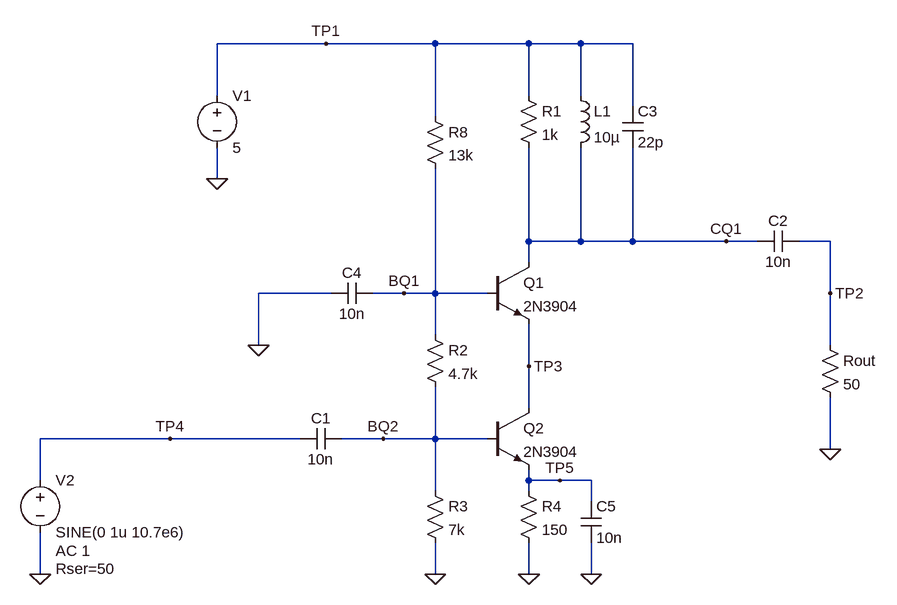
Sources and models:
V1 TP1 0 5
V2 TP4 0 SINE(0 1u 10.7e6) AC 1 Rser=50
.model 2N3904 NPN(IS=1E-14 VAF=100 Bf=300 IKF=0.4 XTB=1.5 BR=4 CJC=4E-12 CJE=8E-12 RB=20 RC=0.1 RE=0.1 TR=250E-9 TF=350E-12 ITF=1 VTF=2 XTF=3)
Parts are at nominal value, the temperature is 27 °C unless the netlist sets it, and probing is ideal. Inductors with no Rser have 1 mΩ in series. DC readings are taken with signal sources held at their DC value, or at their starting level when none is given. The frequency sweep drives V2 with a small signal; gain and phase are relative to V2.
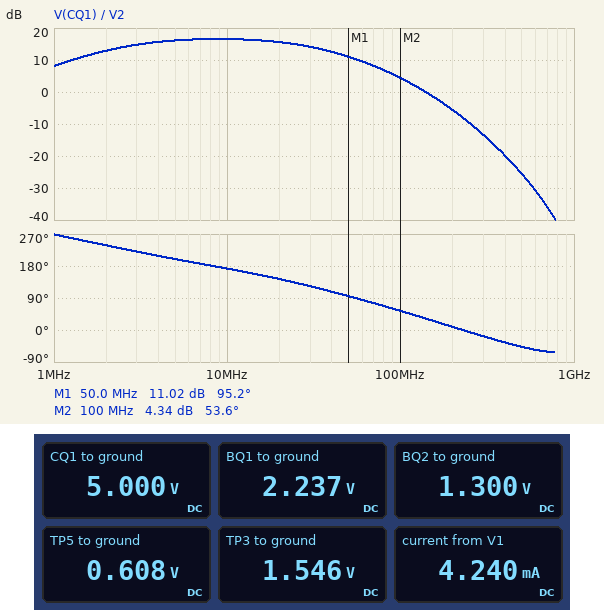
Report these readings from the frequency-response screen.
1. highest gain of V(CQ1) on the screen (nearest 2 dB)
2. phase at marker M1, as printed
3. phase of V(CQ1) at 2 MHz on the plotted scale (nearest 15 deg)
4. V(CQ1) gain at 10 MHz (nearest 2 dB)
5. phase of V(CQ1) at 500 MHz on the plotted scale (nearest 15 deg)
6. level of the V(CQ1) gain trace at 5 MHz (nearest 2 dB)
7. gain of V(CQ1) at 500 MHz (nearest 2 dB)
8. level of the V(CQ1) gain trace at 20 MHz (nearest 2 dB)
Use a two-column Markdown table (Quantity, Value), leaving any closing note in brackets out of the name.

| Quantity | Value |
|---|---|
| highest gain of V(CQ1) on the screen | 16 dB |
| phase at marker M1, as printed | 95.2 deg |
| phase of V(CQ1) at 2 MHz on the plotted scale | 240 deg |
| V(CQ1) gain at 10 MHz | 16 dB |
| phase of V(CQ1) at 500 MHz on the plotted scale | -45 deg |
| level of the V(CQ1) gain trace at 5 MHz | 16 dB |
| gain of V(CQ1) at 500 MHz | -26 dB |
| level of the V(CQ1) gain trace at 20 MHz | 16 dB |
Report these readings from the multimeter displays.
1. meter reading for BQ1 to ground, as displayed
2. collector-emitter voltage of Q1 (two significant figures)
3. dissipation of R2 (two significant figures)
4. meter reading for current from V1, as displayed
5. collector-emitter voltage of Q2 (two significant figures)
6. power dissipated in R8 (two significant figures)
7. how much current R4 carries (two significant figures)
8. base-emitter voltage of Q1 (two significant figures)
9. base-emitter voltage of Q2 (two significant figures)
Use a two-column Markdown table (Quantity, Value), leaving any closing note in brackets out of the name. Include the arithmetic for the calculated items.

| Quantity | Value |
|---|---|
| meter reading for BQ1 to ground, as displayed | 2.237 V |
| collector-emitter voltage of Q1 | 5 V - 1.546 V = 3.5 V |
| dissipation of R2 | (2.237 V - 1.3 V)^2 / 4.7 kΩ = 190 µW |
| meter reading for current from V1, as displayed | 4.240 mA |
| collector-emitter voltage of Q2 | 1.546 V - 608 mV = 940 mV |
| power dissipated in R8 | (5 V - 2.237 V)^2 / 13 kΩ = 590 µW |
| how much current R4 carries | (608 mV) / 150 Ω = 4.1 mA |
| base-emitter voltage of Q1 | 2.237 V - 1.546 V = 690 mV |
| base-emitter voltage of Q2 | 1.3 V - 608 mV = 690 mV |
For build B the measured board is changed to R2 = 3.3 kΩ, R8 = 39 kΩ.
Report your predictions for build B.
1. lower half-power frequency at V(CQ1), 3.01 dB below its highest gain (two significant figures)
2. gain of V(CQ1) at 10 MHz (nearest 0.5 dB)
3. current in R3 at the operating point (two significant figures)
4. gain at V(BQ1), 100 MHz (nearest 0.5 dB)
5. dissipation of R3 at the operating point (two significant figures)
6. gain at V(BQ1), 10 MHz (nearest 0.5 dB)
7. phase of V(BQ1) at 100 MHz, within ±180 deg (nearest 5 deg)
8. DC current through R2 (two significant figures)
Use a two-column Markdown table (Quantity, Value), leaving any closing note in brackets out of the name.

| Quantity | Value |
|---|---|
| lower half-power frequency at V(CQ1), 3.01 dB below its highest gain | 560 kHz |
| gain of V(CQ1) at 10 MHz | -3.0 dB |
| current in R3 at the operating point | 99 µA |
| gain at V(BQ1), 100 MHz | -61.0 dB |
| dissipation of R3 at the operating point | 69 µW |
| gain at V(BQ1), 10 MHz | -54.5 dB |
| phase of V(BQ1) at 100 MHz, within ±180 deg | 80 deg |
| DC current through R2 | 100 µA |
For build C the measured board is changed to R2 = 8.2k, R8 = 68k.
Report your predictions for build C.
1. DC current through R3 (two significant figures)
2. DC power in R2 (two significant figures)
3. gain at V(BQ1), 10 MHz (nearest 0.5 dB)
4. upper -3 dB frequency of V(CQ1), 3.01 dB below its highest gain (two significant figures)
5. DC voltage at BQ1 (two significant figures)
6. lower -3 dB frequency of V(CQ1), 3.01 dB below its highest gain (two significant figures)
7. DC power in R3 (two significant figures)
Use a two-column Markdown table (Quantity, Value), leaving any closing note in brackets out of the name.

| Quantity | Value |
|---|---|
| DC current through R3 | 60 µA |
| DC power in R2 | 30 µW |
| gain at V(BQ1), 10 MHz | -69.5 dB |
| upper -3 dB frequency of V(CQ1), 3.01 dB below its highest gain | 2.3 GHz |
| DC voltage at BQ1 | 910 mV |
| lower -3 dB frequency of V(CQ1), 3.01 dB below its highest gain | 210 MHz |
| DC power in R3 | 25 µW |
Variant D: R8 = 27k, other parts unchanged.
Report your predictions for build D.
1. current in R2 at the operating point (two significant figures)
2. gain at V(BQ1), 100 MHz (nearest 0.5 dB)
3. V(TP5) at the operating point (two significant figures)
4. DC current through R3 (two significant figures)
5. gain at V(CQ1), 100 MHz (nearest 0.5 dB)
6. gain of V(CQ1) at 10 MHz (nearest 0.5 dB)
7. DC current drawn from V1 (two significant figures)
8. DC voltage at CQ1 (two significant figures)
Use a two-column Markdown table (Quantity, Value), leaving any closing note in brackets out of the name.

| Quantity | Value |
|---|---|
| current in R2 at the operating point | 130 µA |
| gain at V(BQ1), 100 MHz | -56.0 dB |
| V(TP5) at the operating point | 200 mV |
| DC current through R3 | 120 µA |
| gain at V(CQ1), 100 MHz | -1.0 dB |
| gain of V(CQ1) at 10 MHz | 7.0 dB |
| DC current drawn from V1 | 1.4 mA |
| DC voltage at CQ1 | 5.0 V |
